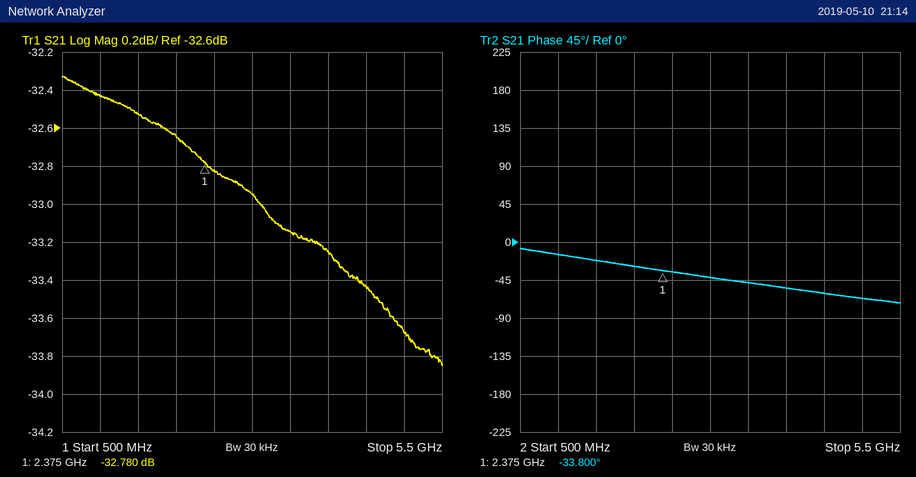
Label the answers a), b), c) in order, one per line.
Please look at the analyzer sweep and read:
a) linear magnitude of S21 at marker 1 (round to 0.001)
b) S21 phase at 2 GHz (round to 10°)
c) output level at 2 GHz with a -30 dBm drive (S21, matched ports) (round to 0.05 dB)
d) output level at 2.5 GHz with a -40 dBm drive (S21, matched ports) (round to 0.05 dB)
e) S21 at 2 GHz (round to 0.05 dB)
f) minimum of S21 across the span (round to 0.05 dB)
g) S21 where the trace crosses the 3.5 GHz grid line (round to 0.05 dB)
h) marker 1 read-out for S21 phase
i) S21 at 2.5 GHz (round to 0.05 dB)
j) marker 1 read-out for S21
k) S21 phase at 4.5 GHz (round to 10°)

a) 0.023
b) -30°
c) -62.65 dBm
d) -72.80 dBm
e) -32.65 dB
f) -33.85 dB
g) -33.15 dB
h) -33.800°
i) -32.80 dB
j) -32.780 dB
k) -60°
